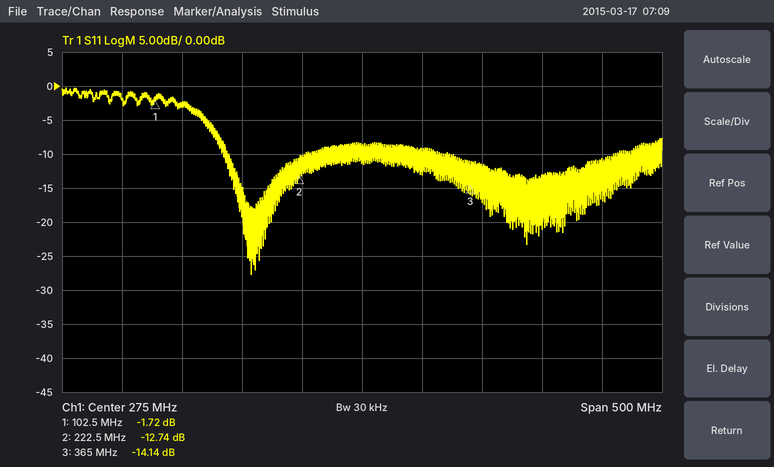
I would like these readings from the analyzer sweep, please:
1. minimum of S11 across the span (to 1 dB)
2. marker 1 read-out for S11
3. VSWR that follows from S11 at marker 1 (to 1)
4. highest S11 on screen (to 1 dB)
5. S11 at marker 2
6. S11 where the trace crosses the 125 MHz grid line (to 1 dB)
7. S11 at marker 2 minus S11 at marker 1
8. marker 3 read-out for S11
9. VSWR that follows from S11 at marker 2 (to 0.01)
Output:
-28 dB
-1.72 dB
10
0 dB
-12.74 dB
-3 dB
-11.02 dB
-14.14 dB
1.60
